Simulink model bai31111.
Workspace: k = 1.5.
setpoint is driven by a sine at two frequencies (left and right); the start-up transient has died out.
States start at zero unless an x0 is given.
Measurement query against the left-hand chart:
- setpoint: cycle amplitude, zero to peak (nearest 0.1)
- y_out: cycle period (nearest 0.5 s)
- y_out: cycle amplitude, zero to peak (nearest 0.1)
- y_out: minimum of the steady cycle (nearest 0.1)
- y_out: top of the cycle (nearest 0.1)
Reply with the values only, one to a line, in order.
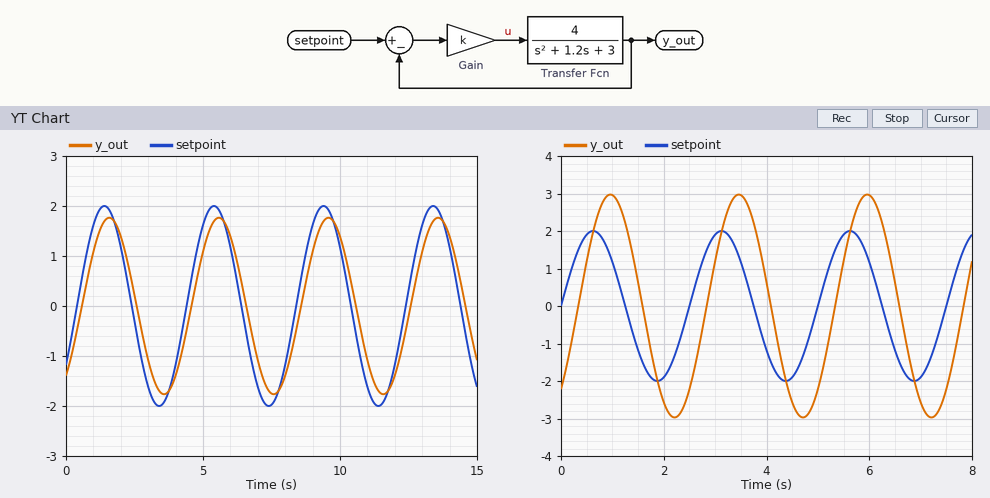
2.0
4.0 s
1.8
-1.8
1.8
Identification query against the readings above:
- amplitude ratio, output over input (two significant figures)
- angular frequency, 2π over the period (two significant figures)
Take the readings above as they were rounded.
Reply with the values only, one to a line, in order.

0.90
1.6 rad/s
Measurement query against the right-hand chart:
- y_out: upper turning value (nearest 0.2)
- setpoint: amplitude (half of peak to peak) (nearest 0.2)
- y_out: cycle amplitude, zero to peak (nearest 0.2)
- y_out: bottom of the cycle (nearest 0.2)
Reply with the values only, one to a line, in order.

3.0
2.0
3.0
-3.0
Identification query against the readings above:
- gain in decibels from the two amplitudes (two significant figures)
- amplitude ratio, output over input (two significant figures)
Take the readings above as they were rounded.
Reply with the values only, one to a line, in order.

3.5 dB
1.5
